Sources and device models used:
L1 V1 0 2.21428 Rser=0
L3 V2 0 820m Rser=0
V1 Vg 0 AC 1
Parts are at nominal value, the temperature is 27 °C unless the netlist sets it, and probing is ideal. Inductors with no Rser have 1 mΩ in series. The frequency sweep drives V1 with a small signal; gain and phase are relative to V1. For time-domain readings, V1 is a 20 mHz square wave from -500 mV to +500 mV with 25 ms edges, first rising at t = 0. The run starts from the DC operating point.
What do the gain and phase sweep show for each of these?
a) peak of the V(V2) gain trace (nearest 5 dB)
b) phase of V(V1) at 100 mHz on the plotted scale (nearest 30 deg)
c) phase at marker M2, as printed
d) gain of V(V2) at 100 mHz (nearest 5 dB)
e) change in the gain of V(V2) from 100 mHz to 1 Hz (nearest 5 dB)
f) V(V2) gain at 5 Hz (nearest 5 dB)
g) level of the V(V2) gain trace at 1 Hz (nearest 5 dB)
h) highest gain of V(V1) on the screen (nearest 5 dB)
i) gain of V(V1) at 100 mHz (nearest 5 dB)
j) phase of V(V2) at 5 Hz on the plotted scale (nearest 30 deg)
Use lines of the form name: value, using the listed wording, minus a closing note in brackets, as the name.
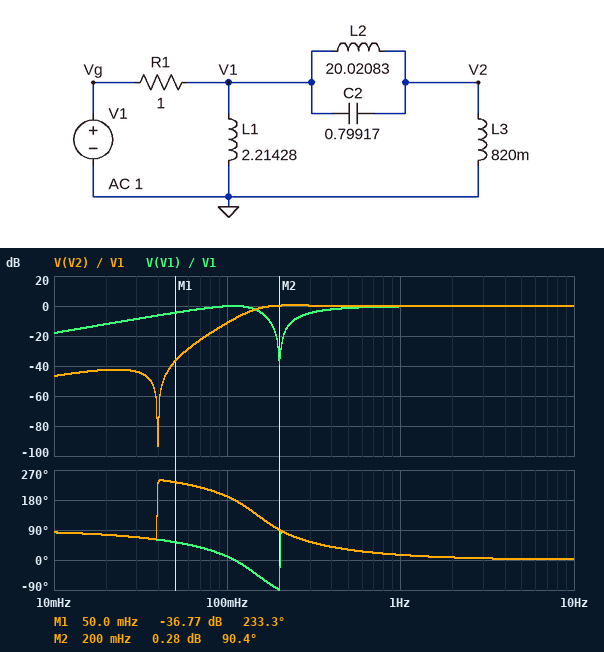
peak of the V(V2) gain trace: 0 dB
phase of V(V1) at 100 mHz on the plotted scale: 0 deg
phase at marker M2, as printed: 90.4 deg
gain of V(V2) at 100 mHz: -10 dB
change in the gain of V(V2) from 100 mHz to 1 Hz: 10 dB
V(V2) gain at 5 Hz: 0 dB
level of the V(V2) gain trace at 1 Hz: 0 dB
highest gain of V(V1) on the screen: 0 dB
gain of V(V1) at 100 mHz: 0 dB
phase of V(V2) at 5 Hz on the plotted scale: 0 deg
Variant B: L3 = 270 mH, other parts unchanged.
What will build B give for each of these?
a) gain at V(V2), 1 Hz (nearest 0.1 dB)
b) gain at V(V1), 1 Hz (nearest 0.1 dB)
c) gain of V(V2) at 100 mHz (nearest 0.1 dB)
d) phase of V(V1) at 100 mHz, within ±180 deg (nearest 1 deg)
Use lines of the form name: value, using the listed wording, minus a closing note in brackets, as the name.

gain at V(V2), 1 Hz: -0.8 dB
gain at V(V1), 1 Hz: -1.9 dB
gain of V(V2) at 100 mHz: -22.5 dB
phase of V(V1) at 100 mHz, within ±180 deg: 15 deg
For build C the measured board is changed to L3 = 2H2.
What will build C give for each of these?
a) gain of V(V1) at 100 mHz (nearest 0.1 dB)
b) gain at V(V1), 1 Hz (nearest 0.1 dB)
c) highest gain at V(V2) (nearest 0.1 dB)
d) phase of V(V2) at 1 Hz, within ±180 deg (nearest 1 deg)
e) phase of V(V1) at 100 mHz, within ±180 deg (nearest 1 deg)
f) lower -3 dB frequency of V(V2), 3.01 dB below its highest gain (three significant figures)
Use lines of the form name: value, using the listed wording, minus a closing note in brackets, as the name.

gain of V(V1) at 100 mHz: -0.4 dB
gain at V(V1), 1 Hz: -0.1 dB
highest gain at V(V2): 5.4 dB
phase of V(V2) at 1 Hz, within ±180 deg: 8 deg
phase of V(V1) at 100 mHz, within ±180 deg: -17 deg
lower -3 dB frequency of V(V2), 3.01 dB below its highest gain: 99.5 mHz
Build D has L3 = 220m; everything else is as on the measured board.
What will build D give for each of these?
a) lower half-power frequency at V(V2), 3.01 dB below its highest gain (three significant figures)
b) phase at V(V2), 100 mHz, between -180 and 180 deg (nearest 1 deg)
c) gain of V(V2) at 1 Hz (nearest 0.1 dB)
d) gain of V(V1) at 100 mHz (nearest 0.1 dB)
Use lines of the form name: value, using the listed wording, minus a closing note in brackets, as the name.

lower half-power frequency at V(V2), 3.01 dB below its highest gain: 597 mHz
phase at V(V2), 100 mHz, between -180 and 180 deg: -165 deg
gain of V(V2) at 1 Hz: -1.3 dB
gain of V(V1) at 100 mHz: -0.3 dB
